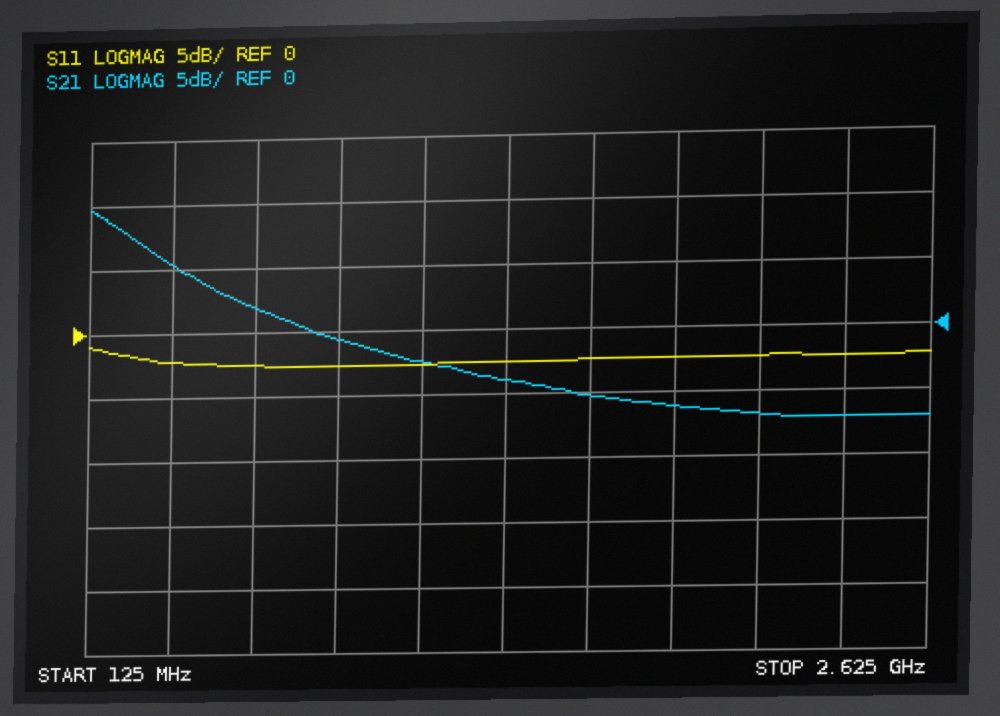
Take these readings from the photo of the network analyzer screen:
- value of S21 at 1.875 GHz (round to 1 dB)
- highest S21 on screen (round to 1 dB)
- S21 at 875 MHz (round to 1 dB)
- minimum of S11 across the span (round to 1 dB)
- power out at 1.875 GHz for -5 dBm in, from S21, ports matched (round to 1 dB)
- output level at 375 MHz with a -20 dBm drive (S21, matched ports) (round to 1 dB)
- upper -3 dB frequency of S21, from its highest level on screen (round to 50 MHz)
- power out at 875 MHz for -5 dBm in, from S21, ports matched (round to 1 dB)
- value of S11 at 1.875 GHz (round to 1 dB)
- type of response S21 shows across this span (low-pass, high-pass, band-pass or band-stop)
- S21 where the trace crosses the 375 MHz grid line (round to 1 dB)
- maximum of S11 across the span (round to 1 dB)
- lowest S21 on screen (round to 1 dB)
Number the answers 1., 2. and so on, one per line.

1. -6 dB
2. 10 dB
3. -1 dB
4. -3 dB
5. -11 dBm
6. -15 dBm
7. 300 MHz
8. -6 dBm
9. -2 dB
10. low-pass
11. 5 dB
12. -1 dB
13. -7 dB
